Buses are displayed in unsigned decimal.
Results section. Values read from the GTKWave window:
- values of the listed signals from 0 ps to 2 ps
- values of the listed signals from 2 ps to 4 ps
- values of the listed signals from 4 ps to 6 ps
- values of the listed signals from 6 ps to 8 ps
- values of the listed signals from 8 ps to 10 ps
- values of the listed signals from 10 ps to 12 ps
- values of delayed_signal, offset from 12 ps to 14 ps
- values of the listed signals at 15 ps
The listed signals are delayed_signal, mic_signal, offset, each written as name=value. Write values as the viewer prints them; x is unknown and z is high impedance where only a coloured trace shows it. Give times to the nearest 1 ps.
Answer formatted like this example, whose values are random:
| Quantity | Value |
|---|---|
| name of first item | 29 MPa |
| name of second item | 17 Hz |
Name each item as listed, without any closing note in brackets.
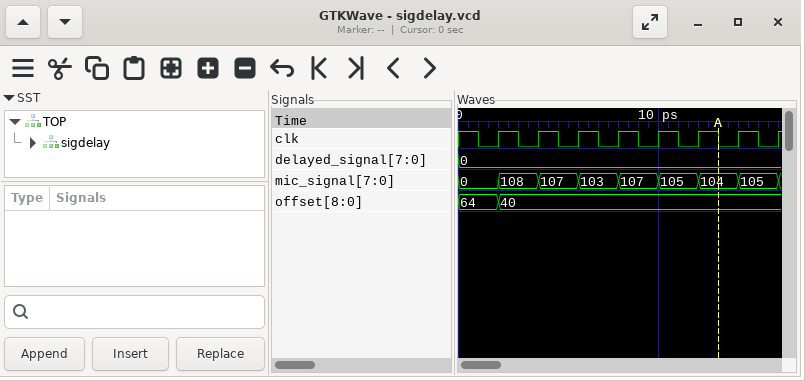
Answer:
| Quantity | Value |
|---|---|
| values of the listed signals from 0 ps to 2 ps | delayed_signal=0, mic_signal=0, offset=64 |
| values of the listed signals from 2 ps to 4 ps | delayed_signal=0, mic_signal=108, offset=40 |
| values of the listed signals from 4 ps to 6 ps | delayed_signal=0, mic_signal=107, offset=40 |
| values of the listed signals from 6 ps to 8 ps | delayed_signal=0, mic_signal=103, offset=40 |
| values of the listed signals from 8 ps to 10 ps | delayed_signal=0, mic_signal=107, offset=40 |
| values of the listed signals from 10 ps to 12 ps | delayed_signal=0, mic_signal=105, offset=40 |
| values of delayed_signal, offset from 12 ps to 14 ps | delayed_signal=0, offset=40 |
| values of the listed signals at 15 ps | delayed_signal=0, mic_signal=105, offset=40 |
